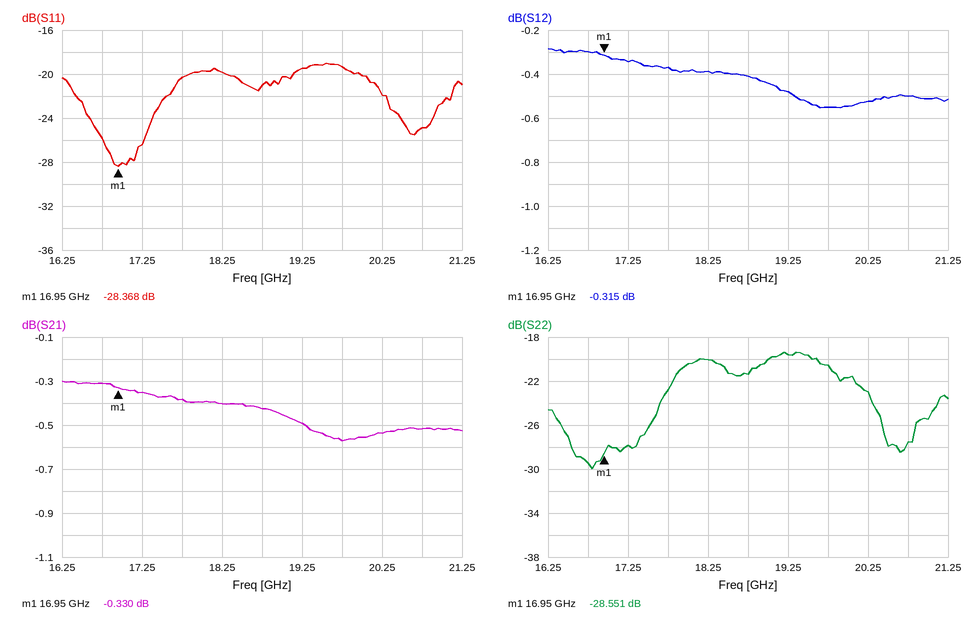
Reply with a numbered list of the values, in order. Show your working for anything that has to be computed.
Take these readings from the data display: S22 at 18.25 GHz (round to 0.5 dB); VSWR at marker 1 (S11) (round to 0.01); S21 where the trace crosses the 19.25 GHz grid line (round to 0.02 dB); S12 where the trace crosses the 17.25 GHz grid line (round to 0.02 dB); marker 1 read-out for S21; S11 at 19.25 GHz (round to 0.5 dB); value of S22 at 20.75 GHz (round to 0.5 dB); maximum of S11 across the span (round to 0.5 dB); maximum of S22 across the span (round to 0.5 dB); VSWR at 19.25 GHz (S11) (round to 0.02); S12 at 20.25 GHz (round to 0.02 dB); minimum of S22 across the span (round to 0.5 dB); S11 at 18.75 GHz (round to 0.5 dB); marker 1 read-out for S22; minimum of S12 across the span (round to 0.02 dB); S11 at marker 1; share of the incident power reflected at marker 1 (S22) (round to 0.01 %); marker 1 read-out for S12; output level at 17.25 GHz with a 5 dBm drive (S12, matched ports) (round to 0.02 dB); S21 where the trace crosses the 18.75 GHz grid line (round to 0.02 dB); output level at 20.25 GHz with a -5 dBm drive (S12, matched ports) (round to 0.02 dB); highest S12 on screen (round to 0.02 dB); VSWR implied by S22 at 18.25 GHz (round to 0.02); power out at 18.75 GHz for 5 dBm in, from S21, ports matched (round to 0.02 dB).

1. -20.0 dB
2. (1 + 0.0382)/(1 − 0.0382) ≈ 1.08
3. -0.50 dB
4. -0.34 dB
5. -0.330 dB
6. -19.5 dB
7. -27.5 dB
8. -19.0 dB
9. -19.5 dB
10. |Γ| = 10^(-19.5/20) = 0.1059; VSWR = (1 + 0.1059)/(1 − 0.1059) ≈ 1.24
11. -0.52 dB
12. -30.0 dB
13. -21.0 dB
14. -28.551 dB
15. -0.56 dB
16. -28.368 dB
17. 10^(-28.551/10) ≈ 0.14 %
18. -0.315 dB
19. 5 dBm + (-0.34 dB) = 4.66 dBm
20. -0.42 dB
21. -5 dBm + (-0.52 dB) = -5.52 dBm
22. -0.28 dB
23. |Γ| = 10^(-20/20) = 0.1000; VSWR = (1 + 0.1000)/(1 − 0.1000) ≈ 1.22
24. 5 dBm + (-0.42 dB) = 4.58 dBm
